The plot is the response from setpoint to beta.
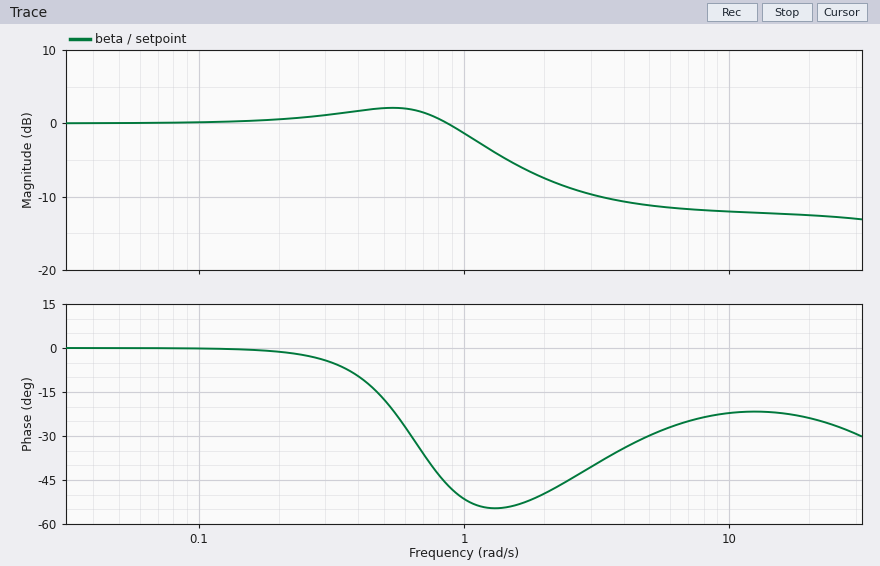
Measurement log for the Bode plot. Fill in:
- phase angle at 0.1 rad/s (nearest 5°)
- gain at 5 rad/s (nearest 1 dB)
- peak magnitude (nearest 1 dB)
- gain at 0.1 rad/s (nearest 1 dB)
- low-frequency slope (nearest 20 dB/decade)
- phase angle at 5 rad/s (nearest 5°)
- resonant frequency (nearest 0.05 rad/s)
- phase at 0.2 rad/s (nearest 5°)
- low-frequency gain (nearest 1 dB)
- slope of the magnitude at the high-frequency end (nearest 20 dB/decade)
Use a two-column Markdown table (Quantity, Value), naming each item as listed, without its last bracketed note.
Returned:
| Quantity | Value |
|---|---|
| phase angle at 0.1 rad/s | 0° |
| gain at 5 rad/s | -11 dB |
| peak magnitude | 2 dB |
| gain at 0.1 rad/s | 0 dB |
| low-frequency slope | 0 dB/decade |
| phase angle at 5 rad/s | -30° |
| resonant frequency | 0.55 rad/s |
| phase at 0.2 rad/s | 0° |
| low-frequency gain | 0 dB |
| slope of the magnitude at the high-frequency end | 0 dB/decade |
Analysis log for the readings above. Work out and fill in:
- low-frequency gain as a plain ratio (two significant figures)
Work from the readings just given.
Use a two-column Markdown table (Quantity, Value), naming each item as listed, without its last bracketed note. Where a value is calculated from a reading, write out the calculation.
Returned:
| Quantity | Value |
|---|---|
| low-frequency gain as a plain ratio | 10^(0 / 20) = 1.0 |
